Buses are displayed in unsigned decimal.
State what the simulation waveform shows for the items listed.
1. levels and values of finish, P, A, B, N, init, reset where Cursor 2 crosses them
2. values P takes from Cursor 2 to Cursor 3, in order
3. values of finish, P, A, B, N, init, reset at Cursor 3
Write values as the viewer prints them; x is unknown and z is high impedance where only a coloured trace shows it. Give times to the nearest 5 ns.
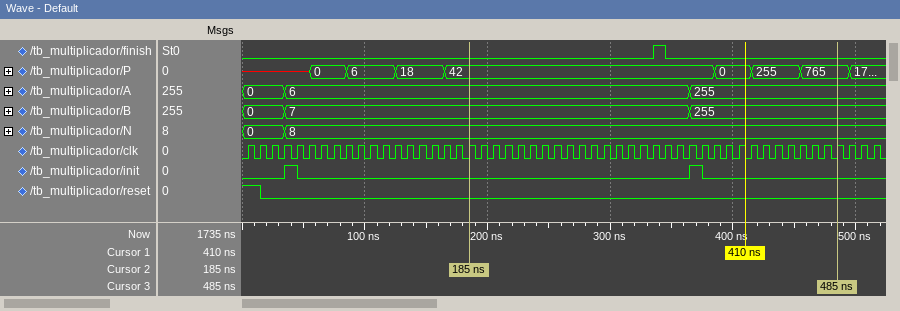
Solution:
finish=0, P=42, A=6, B=7, N=8, init=0, reset=0
42, 0, 255, 765
finish=0, P=765, A=255, B=255, N=8, init=0, reset=0
